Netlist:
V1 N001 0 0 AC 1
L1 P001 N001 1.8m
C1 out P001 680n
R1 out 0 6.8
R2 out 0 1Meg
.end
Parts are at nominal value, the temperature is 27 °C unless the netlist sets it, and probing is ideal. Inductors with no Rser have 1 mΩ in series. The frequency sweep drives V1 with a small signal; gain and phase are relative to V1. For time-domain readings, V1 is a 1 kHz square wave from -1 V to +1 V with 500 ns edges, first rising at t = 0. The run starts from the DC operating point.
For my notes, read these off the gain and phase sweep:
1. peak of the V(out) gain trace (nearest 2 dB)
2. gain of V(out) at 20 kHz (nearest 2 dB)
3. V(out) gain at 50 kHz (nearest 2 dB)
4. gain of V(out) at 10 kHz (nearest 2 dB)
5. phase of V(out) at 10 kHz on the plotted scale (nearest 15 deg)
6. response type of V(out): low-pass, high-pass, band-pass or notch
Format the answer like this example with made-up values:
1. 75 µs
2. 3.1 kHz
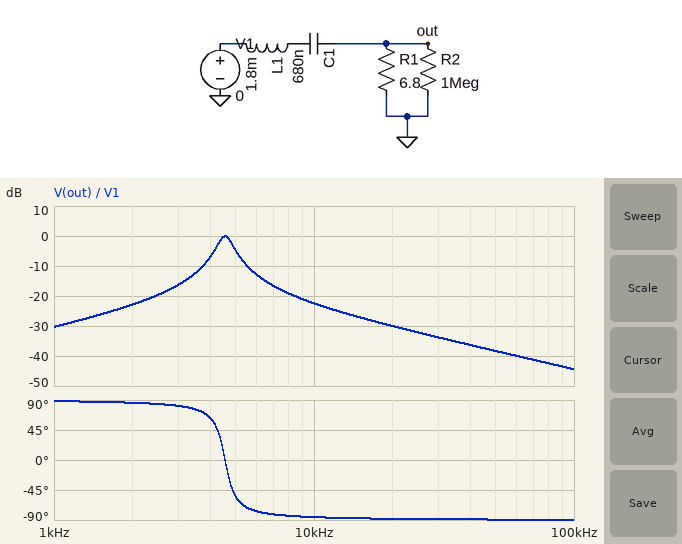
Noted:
1. 0 dB
2. -30 dB
3. -38 dB
4. -22 dB
5. -90 deg
6. band-pass
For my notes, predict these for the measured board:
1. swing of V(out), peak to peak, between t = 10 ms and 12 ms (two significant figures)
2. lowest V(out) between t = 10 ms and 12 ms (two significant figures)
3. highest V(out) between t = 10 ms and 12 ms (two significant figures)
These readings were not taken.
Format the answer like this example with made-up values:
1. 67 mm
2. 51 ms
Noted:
1. 450 mV
2. -230 mV
3. 230 mV
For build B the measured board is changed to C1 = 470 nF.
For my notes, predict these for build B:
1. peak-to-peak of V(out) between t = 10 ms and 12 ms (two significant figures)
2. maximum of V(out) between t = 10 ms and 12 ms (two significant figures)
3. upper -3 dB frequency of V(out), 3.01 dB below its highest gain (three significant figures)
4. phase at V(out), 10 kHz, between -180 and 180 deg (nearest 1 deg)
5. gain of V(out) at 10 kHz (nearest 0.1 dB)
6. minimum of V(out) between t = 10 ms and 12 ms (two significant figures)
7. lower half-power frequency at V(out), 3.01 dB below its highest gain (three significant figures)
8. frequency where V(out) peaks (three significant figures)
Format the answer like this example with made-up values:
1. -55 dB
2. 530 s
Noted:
1. 400 mV
2. 200 mV
3. 5.78 kHz
4. -85 deg
5. -21.4 dB
6. -200 mV
7. 5.18 kHz
8. 5.47 kHz
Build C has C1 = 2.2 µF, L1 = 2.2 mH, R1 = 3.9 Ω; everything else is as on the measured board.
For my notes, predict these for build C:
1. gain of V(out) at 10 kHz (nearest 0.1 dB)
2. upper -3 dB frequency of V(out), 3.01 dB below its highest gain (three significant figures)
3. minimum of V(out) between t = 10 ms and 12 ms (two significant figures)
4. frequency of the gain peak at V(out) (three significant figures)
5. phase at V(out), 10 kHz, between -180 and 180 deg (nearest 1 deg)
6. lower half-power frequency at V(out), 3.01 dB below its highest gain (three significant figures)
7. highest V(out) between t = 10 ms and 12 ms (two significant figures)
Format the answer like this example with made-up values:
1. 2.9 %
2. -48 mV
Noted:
1. -30.5 dB
2. 2.43 kHz
3. -150 mV
4. 2.29 kHz
5. -88 deg
6. 2.15 kHz
7. 150 mV
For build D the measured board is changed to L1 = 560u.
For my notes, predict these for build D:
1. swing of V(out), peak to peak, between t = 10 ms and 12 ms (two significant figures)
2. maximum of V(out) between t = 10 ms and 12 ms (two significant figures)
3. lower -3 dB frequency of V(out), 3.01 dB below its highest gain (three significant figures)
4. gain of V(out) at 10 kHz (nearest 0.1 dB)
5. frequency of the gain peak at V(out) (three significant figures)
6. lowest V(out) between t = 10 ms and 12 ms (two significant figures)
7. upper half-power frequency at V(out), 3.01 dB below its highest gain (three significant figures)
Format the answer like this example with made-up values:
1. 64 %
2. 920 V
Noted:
1. 760 mV
2. 380 mV
3. 7.25 kHz
4. -6.0 dB
5. 8.16 kHz
6. -380 mV
7. 9.18 kHz
